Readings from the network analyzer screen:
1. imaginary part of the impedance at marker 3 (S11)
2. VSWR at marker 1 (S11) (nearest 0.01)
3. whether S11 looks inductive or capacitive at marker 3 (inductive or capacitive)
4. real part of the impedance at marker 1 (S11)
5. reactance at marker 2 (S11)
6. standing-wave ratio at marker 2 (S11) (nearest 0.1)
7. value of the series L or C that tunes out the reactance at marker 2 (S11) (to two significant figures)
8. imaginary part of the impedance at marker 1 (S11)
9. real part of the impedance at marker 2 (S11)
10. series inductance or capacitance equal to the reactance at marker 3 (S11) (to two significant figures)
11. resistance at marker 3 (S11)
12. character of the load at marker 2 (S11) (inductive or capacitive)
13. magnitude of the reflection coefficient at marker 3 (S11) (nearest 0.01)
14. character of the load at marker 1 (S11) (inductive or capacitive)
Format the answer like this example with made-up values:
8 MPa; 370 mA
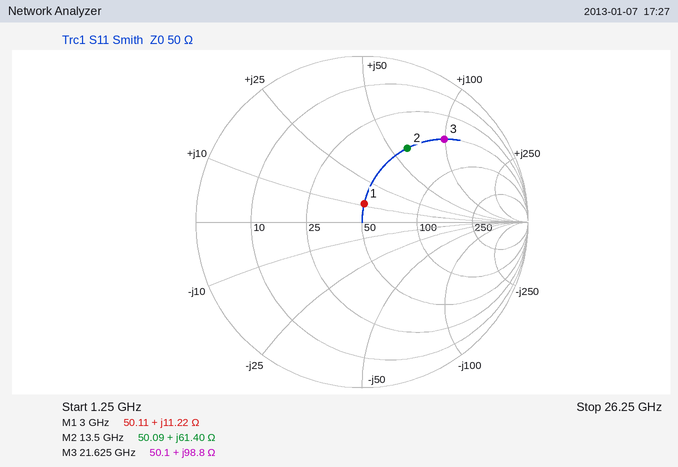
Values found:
+98.8 Ω; 1.25; inductive; 50.11 Ω; +61.40 Ω; 3.2; 190 fF; +11.22 Ω; 50.09 Ω; 730 pH; 50.1 Ω; inductive; 0.70; inductive
